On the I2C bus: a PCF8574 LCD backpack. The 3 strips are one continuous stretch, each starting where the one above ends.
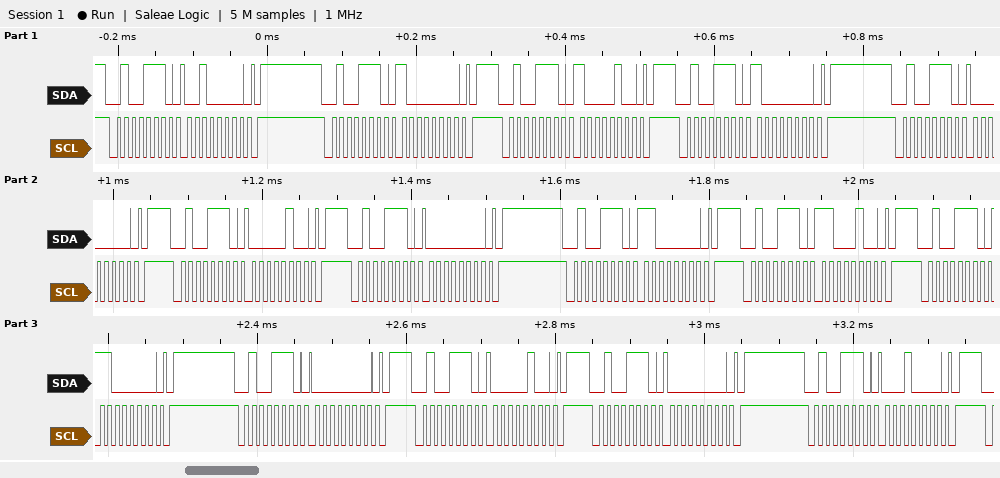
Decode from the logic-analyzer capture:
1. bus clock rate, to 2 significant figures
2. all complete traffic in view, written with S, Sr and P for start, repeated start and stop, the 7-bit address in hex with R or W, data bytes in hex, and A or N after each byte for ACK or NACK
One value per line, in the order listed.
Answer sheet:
100 kHz
S 27W A 20 A P S 27W A 80 A P S 27W A 84 A P S 27W A 80 A P S 27W A 00 A P S 27W A 04 A P S 27W A 00 A P S 27W A C0 A P S 27W A C4 A P S 27W A C0 A P S 27W A 00 A P S 27W A 04 A P S 27W A 00 A P S 27W A 10 A P
